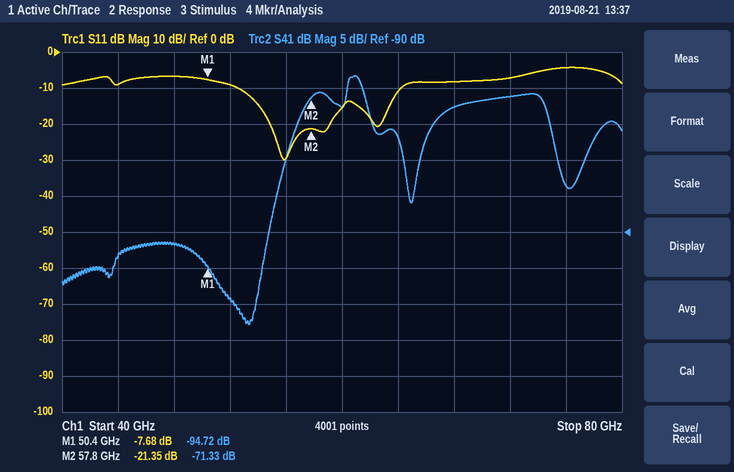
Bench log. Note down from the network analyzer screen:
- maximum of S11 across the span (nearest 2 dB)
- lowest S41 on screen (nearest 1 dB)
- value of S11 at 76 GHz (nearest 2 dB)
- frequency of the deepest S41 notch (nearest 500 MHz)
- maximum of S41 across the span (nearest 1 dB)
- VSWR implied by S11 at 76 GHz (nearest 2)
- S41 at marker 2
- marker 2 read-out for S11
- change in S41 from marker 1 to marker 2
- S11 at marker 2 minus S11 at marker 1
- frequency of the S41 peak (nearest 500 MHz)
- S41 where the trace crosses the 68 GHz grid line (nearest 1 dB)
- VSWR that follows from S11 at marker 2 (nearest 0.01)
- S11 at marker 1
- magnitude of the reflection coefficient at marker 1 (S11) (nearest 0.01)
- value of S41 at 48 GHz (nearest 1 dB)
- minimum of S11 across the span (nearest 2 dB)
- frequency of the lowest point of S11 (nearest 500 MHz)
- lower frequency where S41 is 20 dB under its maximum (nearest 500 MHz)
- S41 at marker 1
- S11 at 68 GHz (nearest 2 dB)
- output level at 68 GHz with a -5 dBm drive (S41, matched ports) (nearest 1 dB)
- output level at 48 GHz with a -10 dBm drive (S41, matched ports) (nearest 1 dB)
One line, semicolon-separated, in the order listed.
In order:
-4 dB; -103 dB; -4 dB; 53.5 GHz; -68 dB; 4; -71.33 dB; -21.35 dB; 23.39 dB; -13.67 dB; 61.0 GHz; -73 dB; 1.19; -7.68 dB; 0.41; -92 dB; -30 dB; 56.0 GHz; 55.0 GHz; -94.72 dB; -8 dB; -78 dBm; -102 dBm
